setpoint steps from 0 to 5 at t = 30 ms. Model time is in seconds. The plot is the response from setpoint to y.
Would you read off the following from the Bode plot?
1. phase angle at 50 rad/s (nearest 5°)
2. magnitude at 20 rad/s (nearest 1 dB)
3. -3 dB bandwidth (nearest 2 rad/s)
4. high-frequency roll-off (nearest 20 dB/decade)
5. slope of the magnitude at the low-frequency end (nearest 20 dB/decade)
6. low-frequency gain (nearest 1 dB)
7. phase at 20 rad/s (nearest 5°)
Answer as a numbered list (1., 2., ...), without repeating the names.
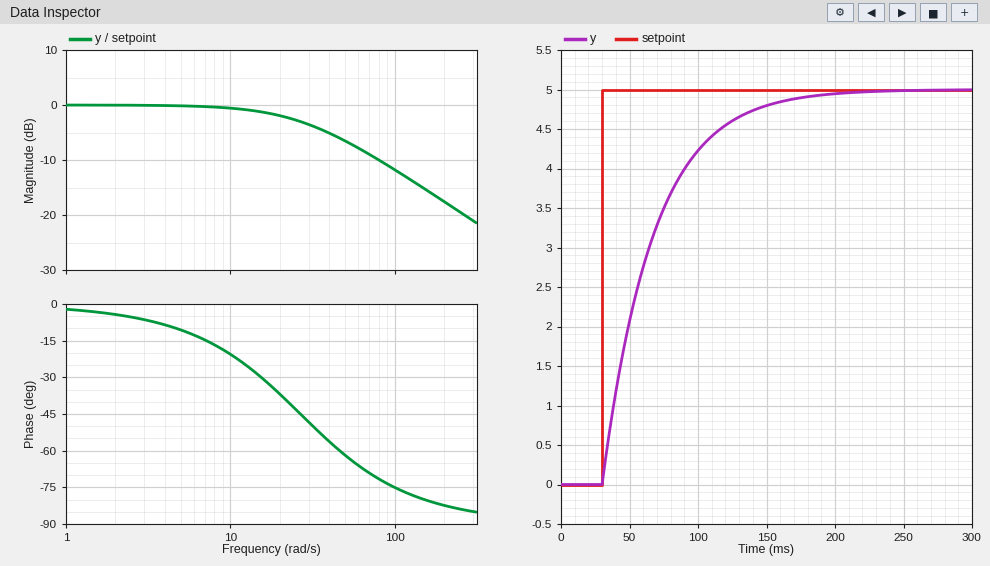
1. -60°
2. -2 dB
3. 26 rad/s
4. -20 dB/decade
5. 0 dB/decade
6. 0 dB
7. -35°
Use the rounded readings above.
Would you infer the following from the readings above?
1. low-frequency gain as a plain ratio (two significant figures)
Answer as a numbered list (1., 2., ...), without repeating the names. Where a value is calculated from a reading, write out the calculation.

1. 10^(0 / 20) = 1.0
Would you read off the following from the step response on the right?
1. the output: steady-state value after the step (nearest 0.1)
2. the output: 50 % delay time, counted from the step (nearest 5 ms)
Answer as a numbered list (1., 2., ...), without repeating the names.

1. 5.0
2. 25 ms
